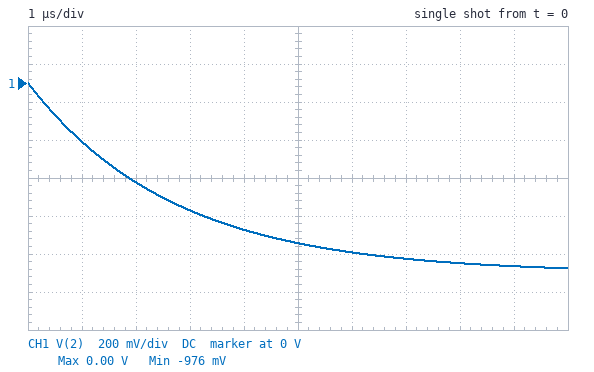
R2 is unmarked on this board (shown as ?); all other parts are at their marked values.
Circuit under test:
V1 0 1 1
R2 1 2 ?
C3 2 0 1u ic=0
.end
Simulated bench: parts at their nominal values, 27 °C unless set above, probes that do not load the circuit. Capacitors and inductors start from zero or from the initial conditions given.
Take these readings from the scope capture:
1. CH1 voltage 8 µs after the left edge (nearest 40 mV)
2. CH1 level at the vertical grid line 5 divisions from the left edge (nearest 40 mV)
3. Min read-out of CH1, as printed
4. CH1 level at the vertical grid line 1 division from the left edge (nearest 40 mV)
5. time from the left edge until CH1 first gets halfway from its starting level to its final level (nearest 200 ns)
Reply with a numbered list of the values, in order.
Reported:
1. -960 mV
2. -840 mV
3. -976 mV
4. -320 mV
5. 1.8 µs
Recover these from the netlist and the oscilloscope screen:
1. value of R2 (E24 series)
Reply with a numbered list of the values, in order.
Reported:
1. 2.7 Ω
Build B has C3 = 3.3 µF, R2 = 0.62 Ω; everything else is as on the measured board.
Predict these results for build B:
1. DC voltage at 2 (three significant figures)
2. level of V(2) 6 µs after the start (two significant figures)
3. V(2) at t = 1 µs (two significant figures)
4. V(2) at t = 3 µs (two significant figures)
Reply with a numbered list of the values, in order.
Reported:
1. -1.00 V
2. -950 mV
3. -390 mV
4. -770 mV
